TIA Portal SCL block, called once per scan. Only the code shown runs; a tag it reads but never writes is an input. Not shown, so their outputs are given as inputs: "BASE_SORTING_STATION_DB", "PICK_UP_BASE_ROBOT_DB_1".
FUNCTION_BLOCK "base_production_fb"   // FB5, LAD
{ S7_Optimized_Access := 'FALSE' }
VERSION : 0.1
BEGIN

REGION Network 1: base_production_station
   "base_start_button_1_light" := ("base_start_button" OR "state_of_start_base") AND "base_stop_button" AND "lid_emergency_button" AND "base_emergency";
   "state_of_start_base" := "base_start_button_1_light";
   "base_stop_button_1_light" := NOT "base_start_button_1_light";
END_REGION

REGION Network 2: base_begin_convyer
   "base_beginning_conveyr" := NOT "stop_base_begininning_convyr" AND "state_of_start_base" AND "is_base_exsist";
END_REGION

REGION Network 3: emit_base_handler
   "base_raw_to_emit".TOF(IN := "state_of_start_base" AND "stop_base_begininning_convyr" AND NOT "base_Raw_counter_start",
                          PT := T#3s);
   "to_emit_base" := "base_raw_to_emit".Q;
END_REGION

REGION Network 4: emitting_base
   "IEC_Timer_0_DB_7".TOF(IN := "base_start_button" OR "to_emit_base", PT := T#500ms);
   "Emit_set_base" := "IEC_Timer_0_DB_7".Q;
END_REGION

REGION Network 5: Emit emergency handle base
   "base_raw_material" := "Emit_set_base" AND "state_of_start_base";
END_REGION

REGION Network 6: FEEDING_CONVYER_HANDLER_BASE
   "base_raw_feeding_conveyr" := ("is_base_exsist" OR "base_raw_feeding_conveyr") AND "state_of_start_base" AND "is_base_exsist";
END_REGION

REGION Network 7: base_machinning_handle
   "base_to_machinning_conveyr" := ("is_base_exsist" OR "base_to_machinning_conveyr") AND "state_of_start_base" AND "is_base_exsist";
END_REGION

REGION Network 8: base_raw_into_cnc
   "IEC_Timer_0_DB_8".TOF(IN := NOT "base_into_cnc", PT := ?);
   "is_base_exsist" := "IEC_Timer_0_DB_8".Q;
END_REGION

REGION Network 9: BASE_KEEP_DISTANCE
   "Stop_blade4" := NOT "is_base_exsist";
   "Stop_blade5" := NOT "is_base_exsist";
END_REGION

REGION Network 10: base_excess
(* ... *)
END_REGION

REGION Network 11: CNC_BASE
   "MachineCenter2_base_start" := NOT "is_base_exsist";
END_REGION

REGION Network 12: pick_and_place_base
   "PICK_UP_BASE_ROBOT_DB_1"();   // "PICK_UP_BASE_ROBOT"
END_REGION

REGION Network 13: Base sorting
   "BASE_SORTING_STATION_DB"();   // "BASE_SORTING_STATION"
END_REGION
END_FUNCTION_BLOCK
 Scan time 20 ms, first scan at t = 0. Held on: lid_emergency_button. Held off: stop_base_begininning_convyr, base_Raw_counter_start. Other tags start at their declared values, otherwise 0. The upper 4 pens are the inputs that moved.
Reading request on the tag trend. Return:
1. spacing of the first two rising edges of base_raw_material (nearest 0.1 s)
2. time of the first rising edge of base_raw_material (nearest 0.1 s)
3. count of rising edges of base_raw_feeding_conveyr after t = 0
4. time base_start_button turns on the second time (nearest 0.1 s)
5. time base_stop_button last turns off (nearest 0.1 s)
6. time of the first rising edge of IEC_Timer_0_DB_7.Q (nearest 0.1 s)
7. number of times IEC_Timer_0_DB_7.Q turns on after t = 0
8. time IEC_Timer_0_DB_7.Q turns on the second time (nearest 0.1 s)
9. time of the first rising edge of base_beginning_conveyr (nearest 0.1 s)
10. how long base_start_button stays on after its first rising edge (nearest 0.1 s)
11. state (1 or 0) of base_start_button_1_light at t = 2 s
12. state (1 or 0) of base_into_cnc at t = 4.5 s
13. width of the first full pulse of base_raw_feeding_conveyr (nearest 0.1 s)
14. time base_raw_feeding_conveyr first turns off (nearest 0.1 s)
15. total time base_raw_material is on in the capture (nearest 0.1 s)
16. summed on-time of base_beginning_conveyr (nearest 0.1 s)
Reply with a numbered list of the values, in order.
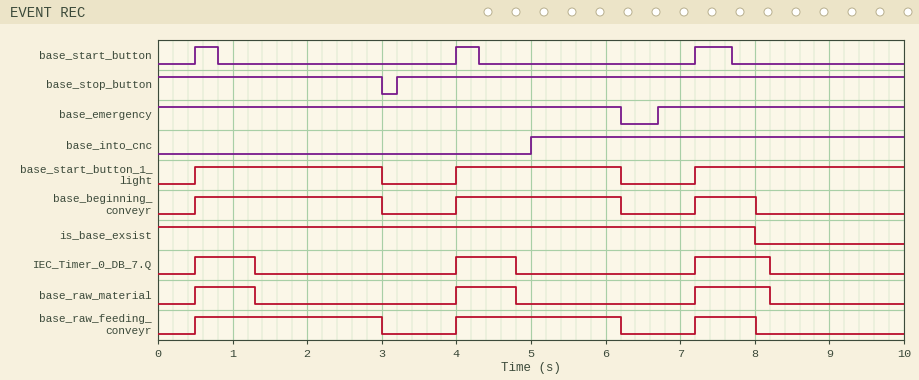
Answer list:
1. 3.5 s
2. 0.5 s
3. 3
4. 4.0 s
5. 3.0 s
6. 0.5 s
7. 3
8. 4.0 s
9. 0.5 s
10. 0.3 s
11. 1
12. 0
13. 2.5 s
14. 3.0 s
15. 2.6 s
16. 5.5 s
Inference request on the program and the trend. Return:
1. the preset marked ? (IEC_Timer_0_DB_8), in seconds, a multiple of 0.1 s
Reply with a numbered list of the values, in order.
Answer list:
1. 3.0 s
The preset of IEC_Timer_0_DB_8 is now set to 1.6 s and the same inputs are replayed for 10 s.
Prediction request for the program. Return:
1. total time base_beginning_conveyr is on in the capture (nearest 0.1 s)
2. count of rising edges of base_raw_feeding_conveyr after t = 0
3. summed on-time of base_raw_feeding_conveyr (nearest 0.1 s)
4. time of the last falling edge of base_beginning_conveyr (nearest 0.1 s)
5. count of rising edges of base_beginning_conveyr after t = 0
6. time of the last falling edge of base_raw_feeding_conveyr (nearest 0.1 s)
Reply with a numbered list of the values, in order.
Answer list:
1. 4.7 s
2. 2
3. 4.7 s
4. 6.2 s
5. 2
6. 6.2 s
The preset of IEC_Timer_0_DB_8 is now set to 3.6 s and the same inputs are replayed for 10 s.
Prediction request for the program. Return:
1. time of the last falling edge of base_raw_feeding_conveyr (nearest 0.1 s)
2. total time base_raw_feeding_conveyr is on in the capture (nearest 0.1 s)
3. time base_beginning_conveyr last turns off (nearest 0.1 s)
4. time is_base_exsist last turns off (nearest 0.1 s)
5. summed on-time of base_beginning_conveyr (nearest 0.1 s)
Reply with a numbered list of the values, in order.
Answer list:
1. 8.6 s
2. 6.1 s
3. 8.6 s
4. 8.6 s
5. 6.1 s
